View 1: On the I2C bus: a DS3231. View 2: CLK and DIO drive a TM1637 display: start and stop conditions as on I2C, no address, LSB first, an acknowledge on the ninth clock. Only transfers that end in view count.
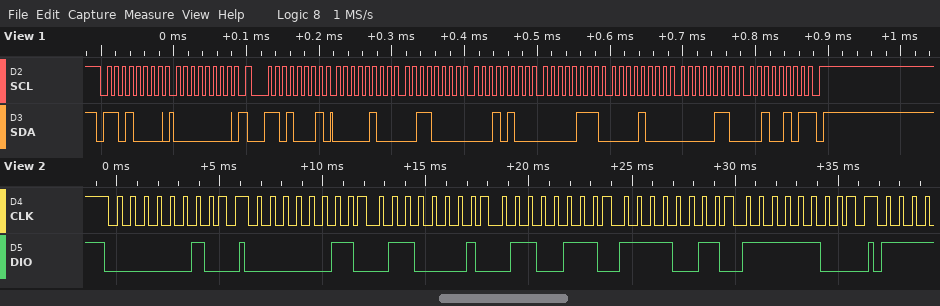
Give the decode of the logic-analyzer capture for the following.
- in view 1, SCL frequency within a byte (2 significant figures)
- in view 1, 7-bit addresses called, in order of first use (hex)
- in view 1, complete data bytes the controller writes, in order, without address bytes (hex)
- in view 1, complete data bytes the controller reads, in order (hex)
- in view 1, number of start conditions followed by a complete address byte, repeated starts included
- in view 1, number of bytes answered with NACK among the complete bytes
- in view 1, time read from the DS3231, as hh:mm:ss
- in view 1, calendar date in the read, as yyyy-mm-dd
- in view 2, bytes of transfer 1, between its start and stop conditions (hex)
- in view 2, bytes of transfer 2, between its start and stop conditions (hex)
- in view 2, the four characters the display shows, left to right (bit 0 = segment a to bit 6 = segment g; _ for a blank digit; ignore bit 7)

100 kHz
0x68
00
04 30 14 07 08 06 25
2
1
14:30:04
2025-06-08
40
C0 86 E6 CF 3F
1430
